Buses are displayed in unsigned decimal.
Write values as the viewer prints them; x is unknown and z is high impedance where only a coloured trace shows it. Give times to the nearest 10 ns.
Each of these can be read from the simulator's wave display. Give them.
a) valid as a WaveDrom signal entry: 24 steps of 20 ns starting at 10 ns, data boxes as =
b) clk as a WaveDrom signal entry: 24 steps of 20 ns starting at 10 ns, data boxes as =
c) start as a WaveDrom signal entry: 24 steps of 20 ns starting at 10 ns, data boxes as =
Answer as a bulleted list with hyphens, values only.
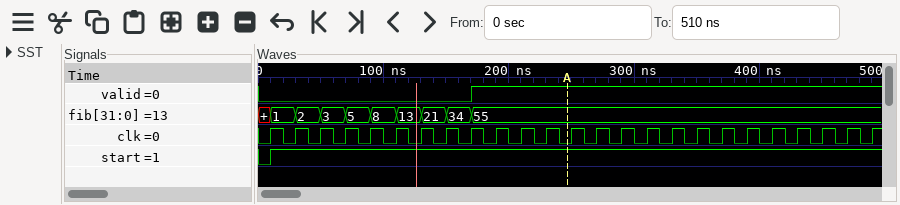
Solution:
- {name: 'valid', wave: '0.......1...............'}
- {name: 'clk', wave: 'p.......................'}
- {name: 'start', wave: '1.......................'}
